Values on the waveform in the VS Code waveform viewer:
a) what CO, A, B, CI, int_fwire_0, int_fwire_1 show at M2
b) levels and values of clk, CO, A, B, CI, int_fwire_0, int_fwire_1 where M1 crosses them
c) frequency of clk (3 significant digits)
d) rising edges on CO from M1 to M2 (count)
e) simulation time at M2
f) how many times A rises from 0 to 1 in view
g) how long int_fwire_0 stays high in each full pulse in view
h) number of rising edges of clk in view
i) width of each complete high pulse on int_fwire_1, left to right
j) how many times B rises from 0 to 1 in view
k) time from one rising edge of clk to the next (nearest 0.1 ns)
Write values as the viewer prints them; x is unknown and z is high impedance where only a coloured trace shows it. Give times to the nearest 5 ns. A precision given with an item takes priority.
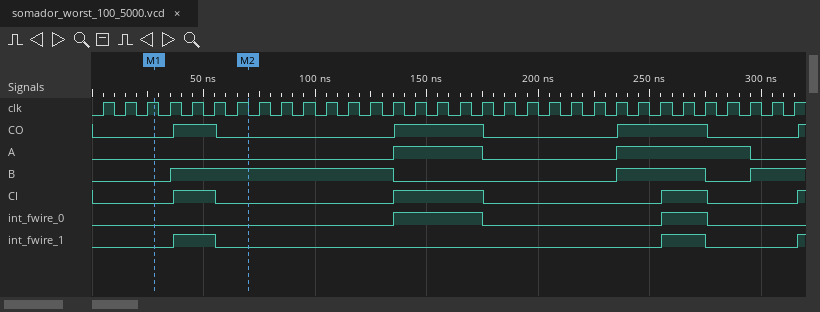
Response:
CO=0, A=0, B=1, CI=0, int_fwire_0=0, int_fwire_1=0
clk=1, CO=0, A=0, B=0, CI=0, int_fwire_0=0, int_fwire_1=0
100 MHz
1
70 ns
2
40 ns, 20 ns
32
20 ns, 20 ns
3
10 ns
